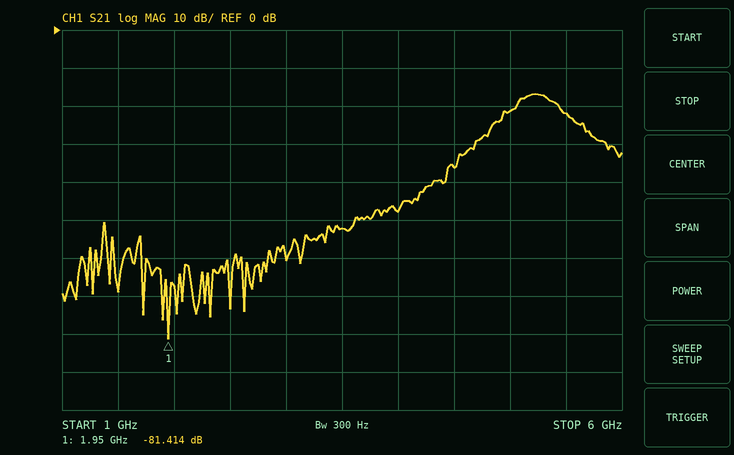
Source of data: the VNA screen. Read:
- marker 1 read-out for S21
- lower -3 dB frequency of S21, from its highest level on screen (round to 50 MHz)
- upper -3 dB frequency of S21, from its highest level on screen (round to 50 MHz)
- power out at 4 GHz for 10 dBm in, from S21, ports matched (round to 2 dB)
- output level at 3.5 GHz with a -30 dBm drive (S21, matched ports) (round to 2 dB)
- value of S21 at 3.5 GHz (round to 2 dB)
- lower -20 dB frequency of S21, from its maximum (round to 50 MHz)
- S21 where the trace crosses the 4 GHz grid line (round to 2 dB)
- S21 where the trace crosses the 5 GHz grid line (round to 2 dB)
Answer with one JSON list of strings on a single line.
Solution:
["-81.414 dB", "5.05 GHz", "5.45 GHz", "-38 dBm", "-82 dBm", "-52 dB", "4.45 GHz", "-48 dB", "-22 dB"]
